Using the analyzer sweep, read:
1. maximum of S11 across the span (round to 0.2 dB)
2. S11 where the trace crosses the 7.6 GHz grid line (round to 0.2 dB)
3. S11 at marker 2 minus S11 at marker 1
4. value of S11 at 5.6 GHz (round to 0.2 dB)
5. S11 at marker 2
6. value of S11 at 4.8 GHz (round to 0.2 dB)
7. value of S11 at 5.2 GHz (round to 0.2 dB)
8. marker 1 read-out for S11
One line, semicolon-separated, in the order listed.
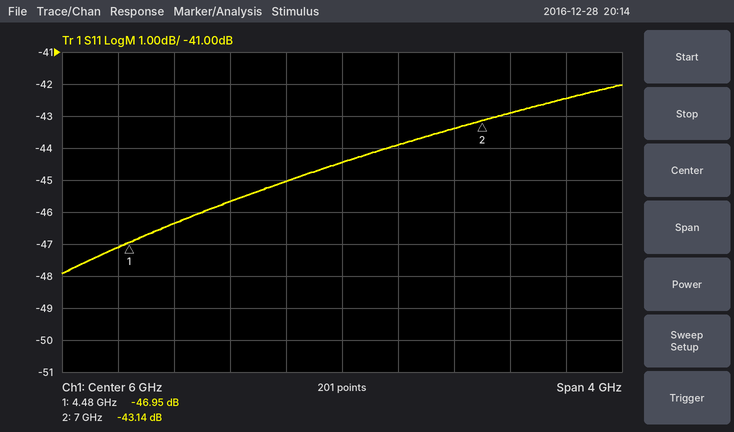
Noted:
-42.0 dB; -42.4 dB; 3.81 dB; -45.0 dB; -43.14 dB; -46.4 dB; -45.6 dB; -46.95 dB
